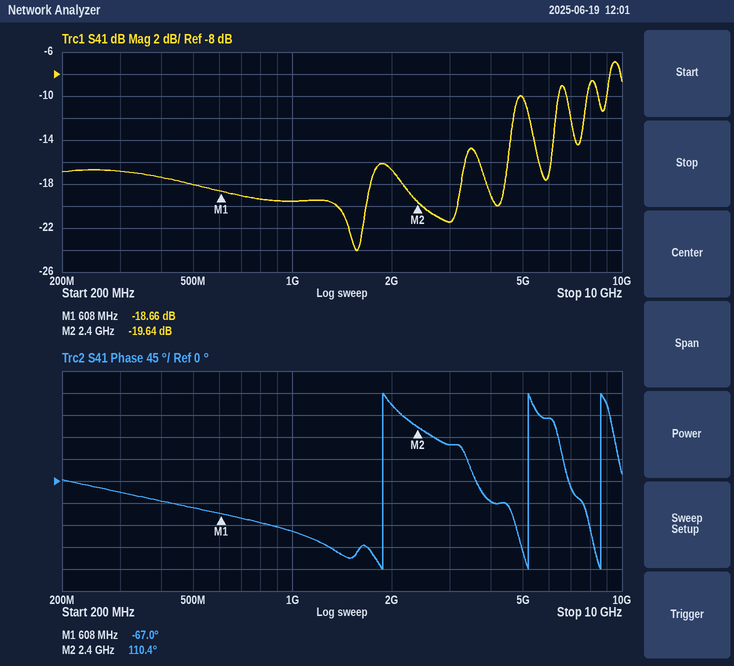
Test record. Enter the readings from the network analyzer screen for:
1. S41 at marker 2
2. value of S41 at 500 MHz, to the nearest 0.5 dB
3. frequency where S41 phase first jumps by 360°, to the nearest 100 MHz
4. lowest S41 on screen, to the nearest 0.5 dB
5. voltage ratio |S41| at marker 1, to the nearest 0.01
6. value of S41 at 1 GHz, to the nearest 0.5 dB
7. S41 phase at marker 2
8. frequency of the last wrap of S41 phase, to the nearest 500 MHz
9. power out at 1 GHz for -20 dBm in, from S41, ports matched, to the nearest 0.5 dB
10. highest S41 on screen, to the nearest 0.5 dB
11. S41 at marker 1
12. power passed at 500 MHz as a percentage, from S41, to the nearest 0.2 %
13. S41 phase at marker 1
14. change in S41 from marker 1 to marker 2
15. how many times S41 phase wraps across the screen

-19.64 dB
-18.0 dB
1.9 GHz
-24.0 dB
0.12
-19.5 dB
110.4°
8.5 GHz
-39.5 dBm
-7.0 dB
-18.66 dB
1.6 %
-67.0°
-0.98 dB
3
